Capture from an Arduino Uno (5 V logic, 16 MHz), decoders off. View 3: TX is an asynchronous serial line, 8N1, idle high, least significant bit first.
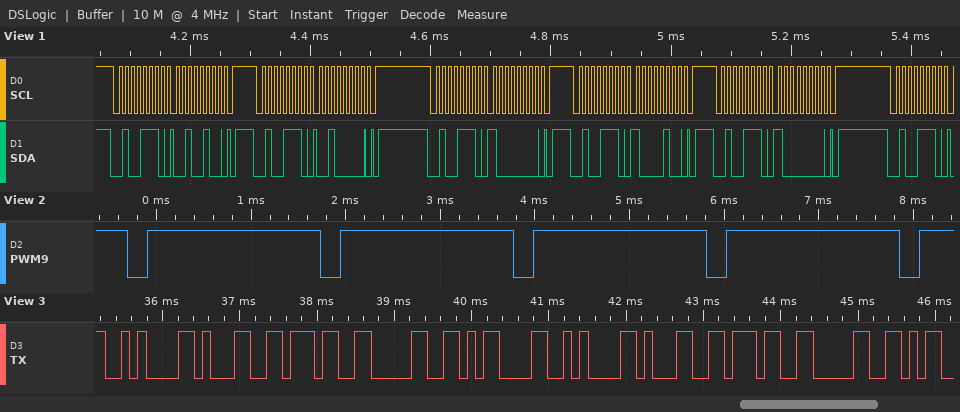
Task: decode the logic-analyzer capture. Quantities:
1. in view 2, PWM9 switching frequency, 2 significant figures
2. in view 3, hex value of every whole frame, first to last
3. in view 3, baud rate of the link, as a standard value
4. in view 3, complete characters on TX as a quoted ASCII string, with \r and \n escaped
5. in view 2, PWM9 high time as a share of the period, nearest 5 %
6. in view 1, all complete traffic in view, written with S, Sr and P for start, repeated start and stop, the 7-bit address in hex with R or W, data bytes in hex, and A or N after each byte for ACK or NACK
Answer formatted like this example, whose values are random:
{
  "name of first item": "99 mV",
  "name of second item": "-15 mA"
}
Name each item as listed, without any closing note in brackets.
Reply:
{
  "in view 2, PWM9 switching frequency, 2 significant figures": "490 Hz",
  "in view 3, hex value of every whole frame, first to last": "0x0A 0x31 0x37 0x30 0x0D 0x0A 0x31 0x37 0x30",
  "in view 3, baud rate of the link, as a standard value": "9600 baud",
  "in view 3, complete characters on TX as a quoted ASCII string, with \\r and \\n escaped": "\"\\n170\\r\\n170\"",
  "in view 2, PWM9 high time as a share of the period, nearest 5 %": "90 %",
  "in view 1, all complete traffic in view, written with S, Sr and P for start, repeated start and stop, the 7-bit address in hex with R or W, data bytes in hex, and A or N after each byte for ACK or NACK": "S 27W A 24 A P S 27W A 20 A P S 27W A 80 A P S 27W A 84 A P S 27W A 80 A P S 27W A"
}
